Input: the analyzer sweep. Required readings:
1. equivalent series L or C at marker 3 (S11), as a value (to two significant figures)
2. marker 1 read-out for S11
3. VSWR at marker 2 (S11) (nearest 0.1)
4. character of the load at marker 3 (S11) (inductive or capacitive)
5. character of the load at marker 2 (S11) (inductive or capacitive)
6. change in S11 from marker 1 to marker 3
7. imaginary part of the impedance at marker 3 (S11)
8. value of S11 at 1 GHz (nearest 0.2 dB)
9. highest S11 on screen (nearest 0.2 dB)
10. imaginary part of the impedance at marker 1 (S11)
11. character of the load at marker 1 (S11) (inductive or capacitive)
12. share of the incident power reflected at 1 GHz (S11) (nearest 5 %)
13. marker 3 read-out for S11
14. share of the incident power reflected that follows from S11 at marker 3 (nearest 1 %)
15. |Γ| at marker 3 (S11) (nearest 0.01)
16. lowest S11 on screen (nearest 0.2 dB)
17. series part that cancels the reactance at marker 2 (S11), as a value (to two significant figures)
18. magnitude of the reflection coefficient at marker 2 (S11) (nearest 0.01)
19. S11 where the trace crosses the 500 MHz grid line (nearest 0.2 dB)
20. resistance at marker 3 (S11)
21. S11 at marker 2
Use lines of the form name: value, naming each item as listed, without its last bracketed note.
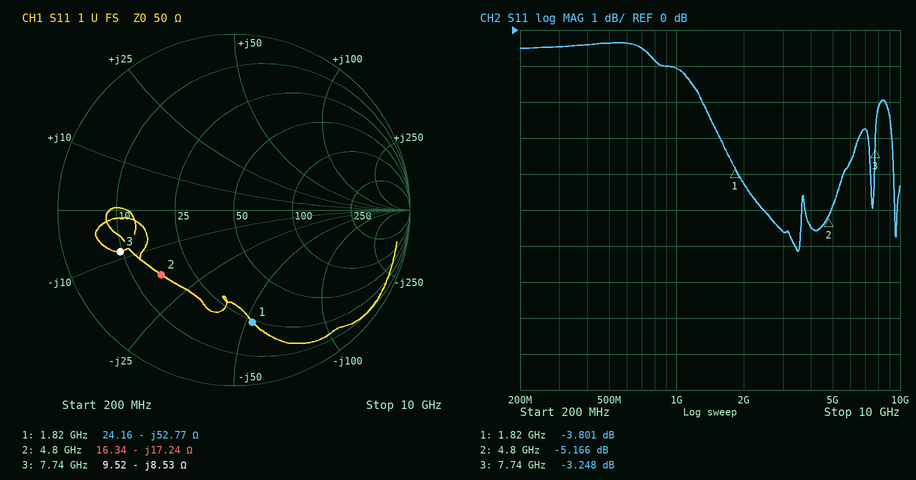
equivalent series L or C at marker 3 (S11), as a value: 2.4 pF
marker 1 read-out for S11: -3.801 dB
VSWR at marker 2 (S11): 3.5
character of the load at marker 3 (S11): capacitive
character of the load at marker 2 (S11): capacitive
change in S11 from marker 1 to marker 3: 0.553 dB
imaginary part of the impedance at marker 3: -8.53 Ω
value of S11 at 1 GHz: -1.0 dB
highest S11 on screen: -0.4 dB
imaginary part of the impedance at marker 1: -52.77 Ω
character of the load at marker 1 (S11): capacitive
share of the incident power reflected at 1 GHz (S11): 80 %
marker 3 read-out for S11: -3.248 dB
share of the incident power reflected that follows from S11 at marker 3: 47 %
|Γ| at marker 3 (S11): 0.69
lowest S11 on screen: -6.2 dB
series part that cancels the reactance at marker 2 (S11), as a value: 570 pH
magnitude of the reflection coefficient at marker 2 (S11): 0.55
S11 where the trace crosses the 500 MHz grid line: -0.4 dB
resistance at marker 3: 9.52 Ω
S11 at marker 2: -5.166 dB
